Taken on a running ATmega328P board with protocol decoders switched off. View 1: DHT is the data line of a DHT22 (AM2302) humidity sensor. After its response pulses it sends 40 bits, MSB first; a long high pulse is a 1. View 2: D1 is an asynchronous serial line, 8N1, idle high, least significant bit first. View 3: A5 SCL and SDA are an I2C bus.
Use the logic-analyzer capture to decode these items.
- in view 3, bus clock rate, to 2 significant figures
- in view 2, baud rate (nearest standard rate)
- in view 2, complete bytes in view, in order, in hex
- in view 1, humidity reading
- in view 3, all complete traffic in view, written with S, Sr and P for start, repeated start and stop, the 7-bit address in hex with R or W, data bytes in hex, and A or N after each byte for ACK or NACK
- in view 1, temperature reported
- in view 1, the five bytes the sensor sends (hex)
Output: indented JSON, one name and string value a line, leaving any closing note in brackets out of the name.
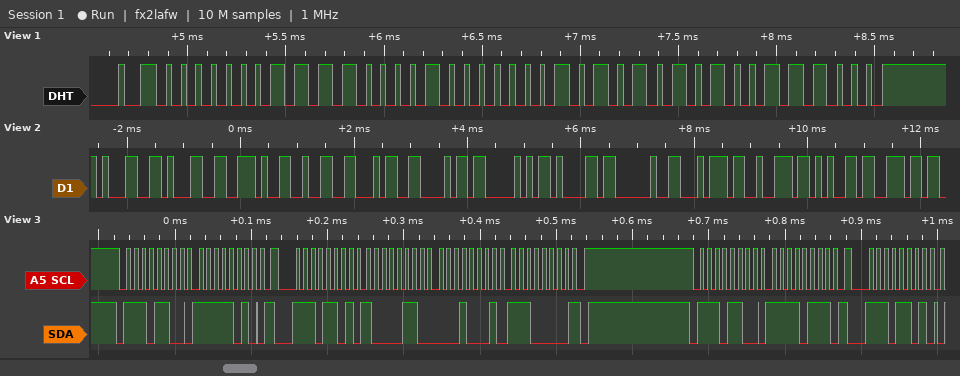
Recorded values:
{
  "in view 3, bus clock rate, to 2 significant figures": "100 kHz",
  "in view 2, baud rate": "9600 baud",
  "in view 2, complete bytes in view, in order, in hex": "31 31 2E 32 34 68 50 61 20 74 72 65 6E",
  "in view 1, humidity reading": "48.1 %",
  "in view 3, all complete traffic in view, written with S, Sr and P for start, repeated start and stop, the 7-bit address in hex with R or W, data bytes in hex, and A or N after each byte for ACK or NACK": "S 76W A FA A Sr 76R A 86 A 11 A E0 N P S 76W A F7 A Sr 76R A",
  "in view 1, temperature reported": "34.1 °C",
  "in view 1, the five bytes the sensor sends": "01 E1 01 55 38"
}
